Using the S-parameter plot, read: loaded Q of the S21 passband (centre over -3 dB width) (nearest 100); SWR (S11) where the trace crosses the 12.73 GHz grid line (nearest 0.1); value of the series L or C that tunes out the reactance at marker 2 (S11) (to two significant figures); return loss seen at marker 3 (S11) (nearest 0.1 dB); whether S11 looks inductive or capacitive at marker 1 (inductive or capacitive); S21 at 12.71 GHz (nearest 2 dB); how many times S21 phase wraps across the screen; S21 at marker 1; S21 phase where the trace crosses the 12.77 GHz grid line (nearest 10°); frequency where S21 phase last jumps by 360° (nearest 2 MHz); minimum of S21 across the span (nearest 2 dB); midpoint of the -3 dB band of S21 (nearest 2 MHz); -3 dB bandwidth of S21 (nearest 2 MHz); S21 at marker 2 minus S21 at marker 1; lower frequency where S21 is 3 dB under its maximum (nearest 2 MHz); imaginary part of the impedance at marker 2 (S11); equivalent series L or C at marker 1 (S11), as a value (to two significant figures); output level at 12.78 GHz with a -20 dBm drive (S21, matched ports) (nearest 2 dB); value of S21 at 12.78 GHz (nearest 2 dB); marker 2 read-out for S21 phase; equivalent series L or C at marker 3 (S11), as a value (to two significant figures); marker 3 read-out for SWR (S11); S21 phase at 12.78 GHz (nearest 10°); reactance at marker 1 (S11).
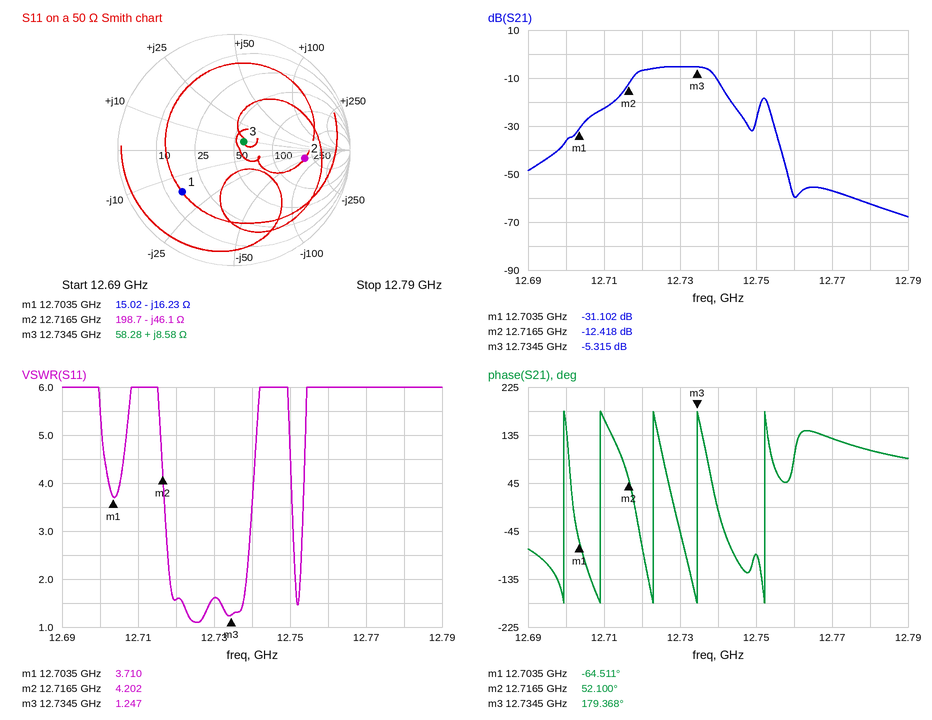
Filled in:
600
1.6
580 pH
19.2 dB
capacitive
-22 dB
5
-31.102 dB
130°
12.752 GHz
-68 dB
12.728 GHz
20 MHz
18.684 dB
12.718 GHz
-46.1 Ω
770 fF
-82 dBm
-62 dB
52.100°
110 pH
1.247
110°
-16.23 Ω
